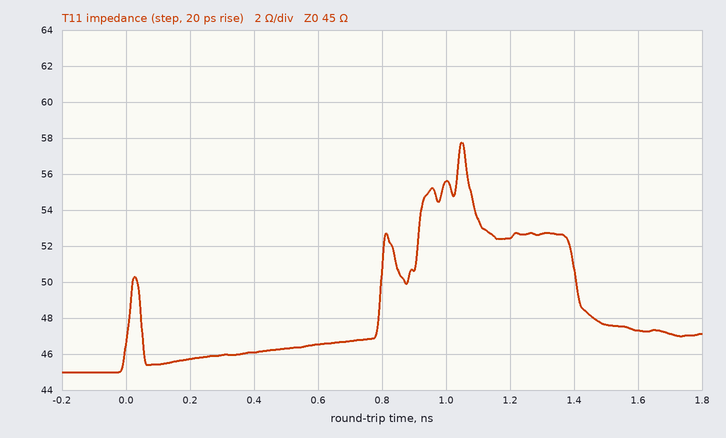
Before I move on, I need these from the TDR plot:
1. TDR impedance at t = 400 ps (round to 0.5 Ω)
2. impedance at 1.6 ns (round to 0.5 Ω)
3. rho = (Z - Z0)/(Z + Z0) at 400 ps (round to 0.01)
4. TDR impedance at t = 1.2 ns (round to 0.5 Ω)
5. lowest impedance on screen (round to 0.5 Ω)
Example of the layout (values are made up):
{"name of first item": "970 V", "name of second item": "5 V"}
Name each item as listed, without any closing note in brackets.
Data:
{"TDR impedance at t = 400 ps": "46.0 Ω", "impedance at 1.6 ns": "47.5 Ω", "rho = (Z - Z0)/(Z + Z0) at 400 ps": "+0.01", "TDR impedance at t = 1.2 ns": "52.5 Ω", "lowest impedance on screen": "45.0 Ω"}
